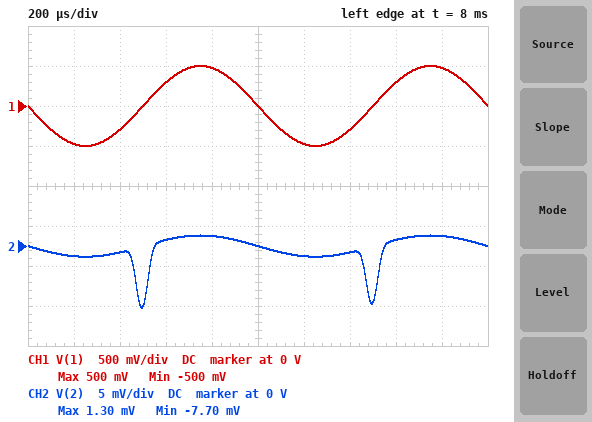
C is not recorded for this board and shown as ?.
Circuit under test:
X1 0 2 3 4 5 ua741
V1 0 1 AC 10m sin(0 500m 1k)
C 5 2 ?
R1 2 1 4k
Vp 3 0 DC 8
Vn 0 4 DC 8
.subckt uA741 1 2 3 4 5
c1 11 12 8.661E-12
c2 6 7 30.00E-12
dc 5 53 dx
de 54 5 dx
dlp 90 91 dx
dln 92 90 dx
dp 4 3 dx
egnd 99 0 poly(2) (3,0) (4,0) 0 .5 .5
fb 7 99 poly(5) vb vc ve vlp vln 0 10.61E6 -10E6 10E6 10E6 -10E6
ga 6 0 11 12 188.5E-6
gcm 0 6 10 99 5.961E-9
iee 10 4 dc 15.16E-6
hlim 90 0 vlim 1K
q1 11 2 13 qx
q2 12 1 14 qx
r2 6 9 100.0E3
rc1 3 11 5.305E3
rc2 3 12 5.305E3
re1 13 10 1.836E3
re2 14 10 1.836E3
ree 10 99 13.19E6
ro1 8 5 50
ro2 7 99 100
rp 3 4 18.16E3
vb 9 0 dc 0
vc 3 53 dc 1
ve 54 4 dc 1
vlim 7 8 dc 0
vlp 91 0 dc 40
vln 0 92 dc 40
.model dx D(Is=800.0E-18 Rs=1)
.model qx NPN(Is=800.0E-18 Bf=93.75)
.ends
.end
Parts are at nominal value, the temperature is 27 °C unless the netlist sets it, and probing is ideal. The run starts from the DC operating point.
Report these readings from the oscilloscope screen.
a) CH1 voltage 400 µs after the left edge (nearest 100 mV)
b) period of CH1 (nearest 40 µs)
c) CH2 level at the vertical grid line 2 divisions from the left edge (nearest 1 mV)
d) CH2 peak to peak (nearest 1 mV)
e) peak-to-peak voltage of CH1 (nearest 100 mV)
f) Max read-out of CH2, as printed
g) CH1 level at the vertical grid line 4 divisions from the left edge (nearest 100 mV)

-300 mV
1.00 ms
-1 mV
9 mV
1.0 V
1.30 mV
500 mV
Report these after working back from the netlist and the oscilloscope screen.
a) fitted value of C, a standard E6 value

15 nF
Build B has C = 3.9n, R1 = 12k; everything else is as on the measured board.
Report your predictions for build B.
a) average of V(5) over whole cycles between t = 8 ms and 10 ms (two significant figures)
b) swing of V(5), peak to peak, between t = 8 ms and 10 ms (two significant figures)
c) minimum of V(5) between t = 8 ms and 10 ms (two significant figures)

5.9 V
3.4 V
4.2 V
